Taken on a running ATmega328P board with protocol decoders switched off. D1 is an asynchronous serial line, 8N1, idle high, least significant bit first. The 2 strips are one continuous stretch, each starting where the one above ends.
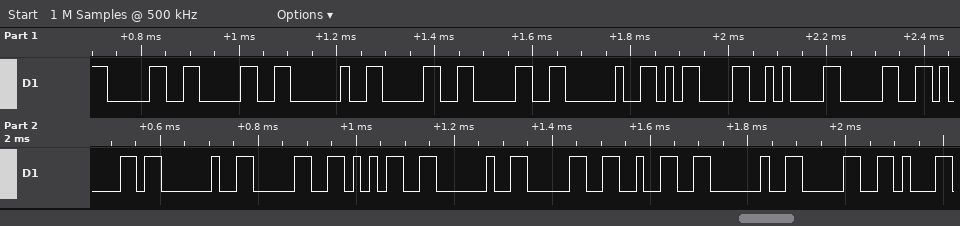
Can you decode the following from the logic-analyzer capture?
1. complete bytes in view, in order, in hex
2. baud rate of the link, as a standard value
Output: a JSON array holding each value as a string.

["30 30 20 30 30 20 0D 0A 30 61 20 30 35 20 30 32 20 30", "57600 baud"]
